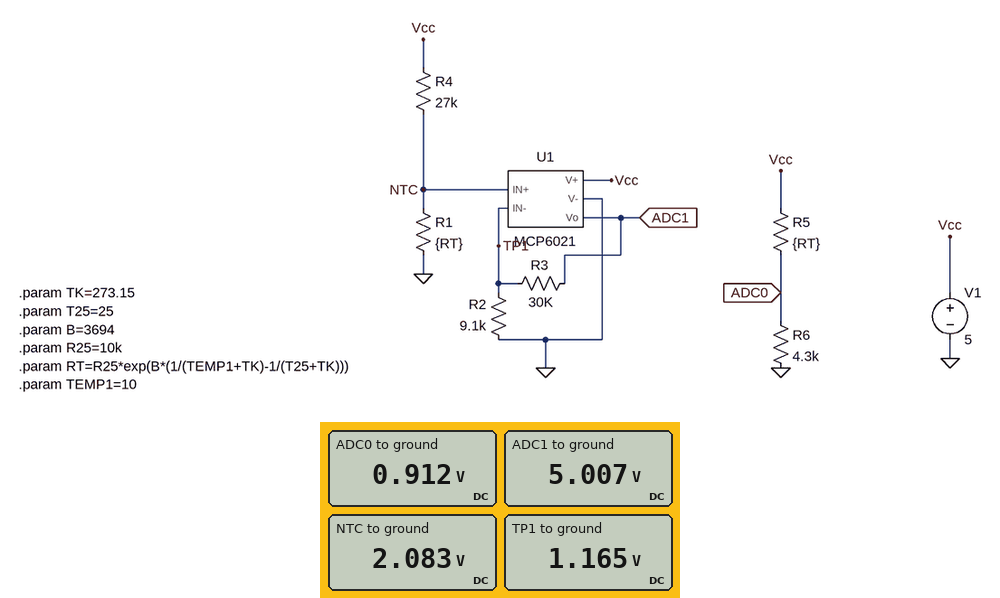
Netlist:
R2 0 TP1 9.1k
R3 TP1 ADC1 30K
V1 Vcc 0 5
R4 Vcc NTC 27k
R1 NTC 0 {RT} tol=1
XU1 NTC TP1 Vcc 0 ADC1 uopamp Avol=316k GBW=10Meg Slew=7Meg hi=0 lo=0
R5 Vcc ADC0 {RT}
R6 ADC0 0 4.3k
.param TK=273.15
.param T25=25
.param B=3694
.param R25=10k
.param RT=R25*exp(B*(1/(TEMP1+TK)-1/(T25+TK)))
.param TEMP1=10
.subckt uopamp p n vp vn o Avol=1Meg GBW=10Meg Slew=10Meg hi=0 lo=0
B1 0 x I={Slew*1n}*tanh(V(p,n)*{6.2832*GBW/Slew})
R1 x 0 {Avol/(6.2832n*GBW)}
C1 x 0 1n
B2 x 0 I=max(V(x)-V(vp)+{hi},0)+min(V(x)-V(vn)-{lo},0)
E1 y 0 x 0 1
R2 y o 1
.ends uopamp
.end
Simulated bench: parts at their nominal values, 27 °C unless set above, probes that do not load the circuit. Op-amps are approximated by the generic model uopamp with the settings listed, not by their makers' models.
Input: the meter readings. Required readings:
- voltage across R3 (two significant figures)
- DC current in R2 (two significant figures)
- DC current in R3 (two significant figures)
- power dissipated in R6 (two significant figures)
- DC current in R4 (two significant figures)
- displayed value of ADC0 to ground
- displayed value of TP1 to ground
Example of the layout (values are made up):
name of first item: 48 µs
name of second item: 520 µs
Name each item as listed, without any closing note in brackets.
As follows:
voltage across R3: 3.8 V
DC current in R2: 130 µA
DC current in R3: 130 µA
power dissipated in R6: 190 µW
DC current in R4: 110 µA
displayed value of ADC0 to ground: 0.912 V
displayed value of TP1 to ground: 1.165 V
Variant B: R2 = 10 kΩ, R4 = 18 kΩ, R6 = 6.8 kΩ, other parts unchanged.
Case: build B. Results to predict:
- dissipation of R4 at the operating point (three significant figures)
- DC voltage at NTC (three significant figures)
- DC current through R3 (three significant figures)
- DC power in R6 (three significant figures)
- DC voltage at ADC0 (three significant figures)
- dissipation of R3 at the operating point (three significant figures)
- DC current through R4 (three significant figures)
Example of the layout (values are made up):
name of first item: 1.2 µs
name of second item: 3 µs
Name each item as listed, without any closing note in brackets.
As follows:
dissipation of R4 at the operating point: 324 µW
DC voltage at NTC: 2.59 V
DC current through R3: 125 µA
DC power in R6: 250 µW
DC voltage at ADC0: 1.30 V
dissipation of R3 at the operating point: 470 µW
DC current through R4: 134 µA
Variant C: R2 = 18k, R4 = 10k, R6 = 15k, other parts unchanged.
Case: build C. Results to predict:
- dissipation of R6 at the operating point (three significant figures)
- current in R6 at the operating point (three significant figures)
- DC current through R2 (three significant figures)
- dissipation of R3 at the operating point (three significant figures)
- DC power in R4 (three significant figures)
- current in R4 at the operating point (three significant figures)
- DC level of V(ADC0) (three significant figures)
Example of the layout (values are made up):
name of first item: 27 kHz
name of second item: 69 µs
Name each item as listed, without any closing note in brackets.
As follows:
dissipation of R6 at the operating point: 319 µW
current in R6 at the operating point: 146 µA
DC current through R2: 104 µA
dissipation of R3 at the operating point: 326 µW
DC power in R4: 292 µW
current in R4 at the operating point: 171 µA
DC level of V(ADC0): 2.19 V
